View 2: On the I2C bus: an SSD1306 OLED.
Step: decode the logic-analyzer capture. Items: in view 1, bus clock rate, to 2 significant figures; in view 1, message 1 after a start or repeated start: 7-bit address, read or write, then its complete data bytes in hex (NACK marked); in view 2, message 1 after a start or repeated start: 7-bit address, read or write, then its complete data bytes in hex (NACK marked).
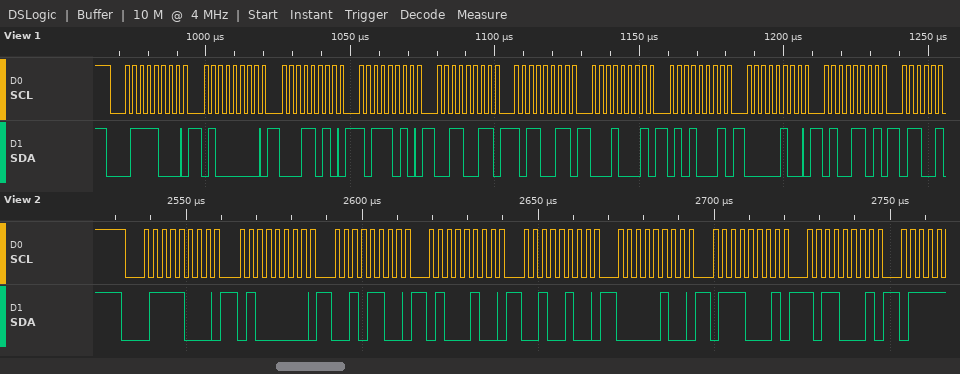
400 kHz
0x3C write: 40 1A BA 33 B3 11 51 04 4D
0x3C write: 40 2C 44 24 04 71 B1
